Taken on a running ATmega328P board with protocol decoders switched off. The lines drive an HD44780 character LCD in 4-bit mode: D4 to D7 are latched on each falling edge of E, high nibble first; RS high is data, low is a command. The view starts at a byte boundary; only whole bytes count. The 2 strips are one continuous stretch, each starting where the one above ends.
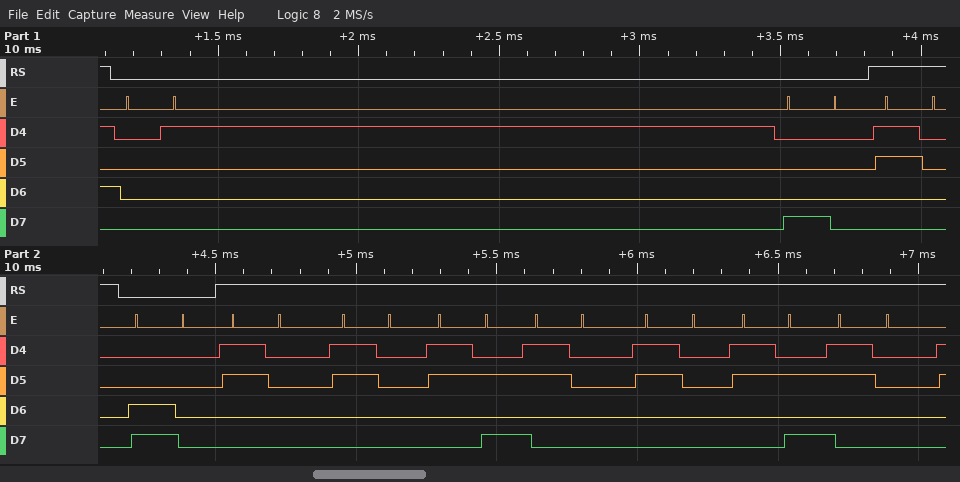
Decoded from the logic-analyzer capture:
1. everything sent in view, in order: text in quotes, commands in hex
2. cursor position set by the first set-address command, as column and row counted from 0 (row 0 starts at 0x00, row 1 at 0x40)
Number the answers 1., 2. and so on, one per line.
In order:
1. 0x01 0x80 "0" 0xC0 "00:00:0"
2. column 0, row 0
